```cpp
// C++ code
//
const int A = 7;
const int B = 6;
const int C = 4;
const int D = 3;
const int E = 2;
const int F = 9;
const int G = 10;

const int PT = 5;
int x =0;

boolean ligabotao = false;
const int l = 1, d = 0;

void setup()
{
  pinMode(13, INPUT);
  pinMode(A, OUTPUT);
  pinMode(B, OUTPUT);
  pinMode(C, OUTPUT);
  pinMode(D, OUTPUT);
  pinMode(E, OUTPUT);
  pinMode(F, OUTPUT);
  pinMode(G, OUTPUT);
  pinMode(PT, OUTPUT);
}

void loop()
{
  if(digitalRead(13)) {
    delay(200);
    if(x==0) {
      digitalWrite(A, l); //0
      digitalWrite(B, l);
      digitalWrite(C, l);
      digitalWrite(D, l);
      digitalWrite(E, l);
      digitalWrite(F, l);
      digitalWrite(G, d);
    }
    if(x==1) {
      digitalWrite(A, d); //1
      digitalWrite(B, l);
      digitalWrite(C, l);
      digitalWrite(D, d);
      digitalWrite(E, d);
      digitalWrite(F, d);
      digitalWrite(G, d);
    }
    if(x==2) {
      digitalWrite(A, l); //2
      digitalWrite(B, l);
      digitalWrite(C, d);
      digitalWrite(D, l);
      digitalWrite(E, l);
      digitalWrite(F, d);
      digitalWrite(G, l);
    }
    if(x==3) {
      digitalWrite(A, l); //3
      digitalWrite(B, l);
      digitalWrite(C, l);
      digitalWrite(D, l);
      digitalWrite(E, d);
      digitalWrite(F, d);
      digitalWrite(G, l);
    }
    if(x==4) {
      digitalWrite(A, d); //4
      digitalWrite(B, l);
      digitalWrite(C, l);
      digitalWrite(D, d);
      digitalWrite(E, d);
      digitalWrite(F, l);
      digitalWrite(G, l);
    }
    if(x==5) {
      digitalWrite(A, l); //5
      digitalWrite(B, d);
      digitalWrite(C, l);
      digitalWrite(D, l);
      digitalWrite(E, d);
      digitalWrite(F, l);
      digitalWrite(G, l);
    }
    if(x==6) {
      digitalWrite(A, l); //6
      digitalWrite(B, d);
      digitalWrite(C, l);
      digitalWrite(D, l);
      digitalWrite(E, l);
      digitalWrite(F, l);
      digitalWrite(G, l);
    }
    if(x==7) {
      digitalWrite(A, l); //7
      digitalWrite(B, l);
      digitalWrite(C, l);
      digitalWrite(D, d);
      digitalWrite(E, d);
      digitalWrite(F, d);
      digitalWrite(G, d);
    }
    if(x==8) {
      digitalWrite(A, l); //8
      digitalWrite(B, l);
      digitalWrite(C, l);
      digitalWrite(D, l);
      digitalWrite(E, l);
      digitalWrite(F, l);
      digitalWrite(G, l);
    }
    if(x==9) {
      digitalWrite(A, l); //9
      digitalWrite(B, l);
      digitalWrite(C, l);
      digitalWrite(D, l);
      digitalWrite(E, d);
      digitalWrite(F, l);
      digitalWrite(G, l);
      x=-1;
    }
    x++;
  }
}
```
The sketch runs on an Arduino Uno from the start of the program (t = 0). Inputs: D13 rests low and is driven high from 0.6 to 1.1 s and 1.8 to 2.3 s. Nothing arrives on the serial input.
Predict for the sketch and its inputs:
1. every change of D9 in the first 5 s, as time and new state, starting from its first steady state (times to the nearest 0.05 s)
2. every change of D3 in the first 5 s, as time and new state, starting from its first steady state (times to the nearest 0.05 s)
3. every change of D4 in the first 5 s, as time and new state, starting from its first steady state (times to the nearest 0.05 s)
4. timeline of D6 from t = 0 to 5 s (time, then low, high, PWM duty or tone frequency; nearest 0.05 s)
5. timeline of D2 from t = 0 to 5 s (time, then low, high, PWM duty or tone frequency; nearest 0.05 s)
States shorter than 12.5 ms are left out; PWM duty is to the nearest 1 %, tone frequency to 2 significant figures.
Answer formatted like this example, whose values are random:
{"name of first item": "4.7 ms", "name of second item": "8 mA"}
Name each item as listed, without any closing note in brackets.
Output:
{"every change of D9 in the first 5 s, as time and new state, starting from its first steady state": "0 s low; 0.8 s high; 1 s low; 2.2 s high", "every change of D3 in the first 5 s, as time and new state, starting from its first steady state": "0 s low; 0.8 s high; 1 s low; 1.2 s high; 2.2 s low; 2.4 s high", "every change of D4 in the first 5 s, as time and new state, starting from its first steady state": "0 s low; 0.8 s high; 1.2 s low; 2 s high", "timeline of D6 from t = 0 to 5 s": "0 s low; 0.8 s high; 2.4 s low", "timeline of D2 from t = 0 to 5 s": "0 s low; 0.8 s high; 1 s low; 1.2 s high; 2 s low"}
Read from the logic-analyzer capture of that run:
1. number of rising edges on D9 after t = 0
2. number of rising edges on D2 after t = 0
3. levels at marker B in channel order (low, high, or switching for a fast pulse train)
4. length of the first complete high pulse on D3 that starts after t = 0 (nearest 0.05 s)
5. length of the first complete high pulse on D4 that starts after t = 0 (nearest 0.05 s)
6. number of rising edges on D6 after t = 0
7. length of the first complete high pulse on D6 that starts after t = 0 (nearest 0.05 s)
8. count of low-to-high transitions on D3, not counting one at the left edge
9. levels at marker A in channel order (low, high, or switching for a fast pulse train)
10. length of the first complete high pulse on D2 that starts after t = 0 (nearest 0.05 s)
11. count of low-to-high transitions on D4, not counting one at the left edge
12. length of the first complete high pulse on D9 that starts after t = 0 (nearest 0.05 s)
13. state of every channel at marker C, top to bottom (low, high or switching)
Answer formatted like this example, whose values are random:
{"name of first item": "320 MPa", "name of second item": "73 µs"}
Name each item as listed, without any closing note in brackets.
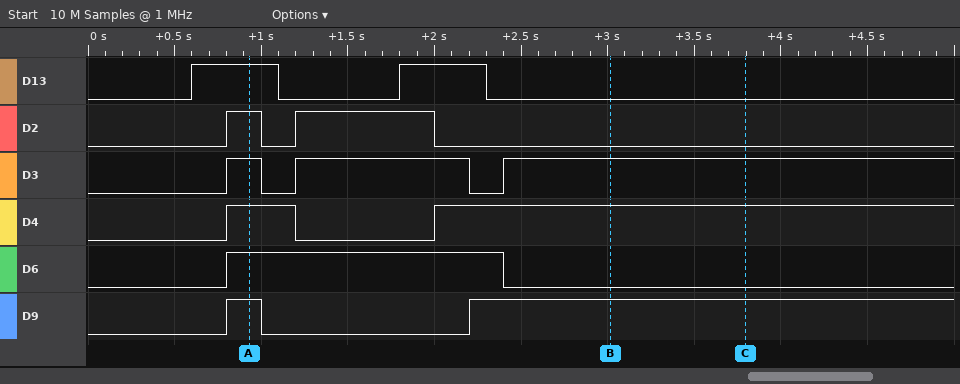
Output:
{"number of rising edges on D9 after t = 0": "2", "number of rising edges on D2 after t = 0": "2", "levels at marker B in channel order": "D13 low, D2 low, D3 high, D4 high, D6 low, D9 high", "length of the first complete high pulse on D3 that starts after t = 0": "0.20 s", "length of the first complete high pulse on D4 that starts after t = 0": "0.40 s", "number of rising edges on D6 after t = 0": "1", "length of the first complete high pulse on D6 that starts after t = 0": "1.60 s", "count of low-to-high transitions on D3, not counting one at the left edge": "3", "levels at marker A in channel order": "D13 high, D2 high, D3 high, D4 high, D6 high, D9 high", "length of the first complete high pulse on D2 that starts after t = 0": "0.20 s", "count of low-to-high transitions on D4, not counting one at the left edge": "2", "length of the first complete high pulse on D9 that starts after t = 0": "0.20 s", "state of every channel at marker C, top to bottom": "D13 low, D2 low, D3 high, D4 high, D6 low, D9 high"}
